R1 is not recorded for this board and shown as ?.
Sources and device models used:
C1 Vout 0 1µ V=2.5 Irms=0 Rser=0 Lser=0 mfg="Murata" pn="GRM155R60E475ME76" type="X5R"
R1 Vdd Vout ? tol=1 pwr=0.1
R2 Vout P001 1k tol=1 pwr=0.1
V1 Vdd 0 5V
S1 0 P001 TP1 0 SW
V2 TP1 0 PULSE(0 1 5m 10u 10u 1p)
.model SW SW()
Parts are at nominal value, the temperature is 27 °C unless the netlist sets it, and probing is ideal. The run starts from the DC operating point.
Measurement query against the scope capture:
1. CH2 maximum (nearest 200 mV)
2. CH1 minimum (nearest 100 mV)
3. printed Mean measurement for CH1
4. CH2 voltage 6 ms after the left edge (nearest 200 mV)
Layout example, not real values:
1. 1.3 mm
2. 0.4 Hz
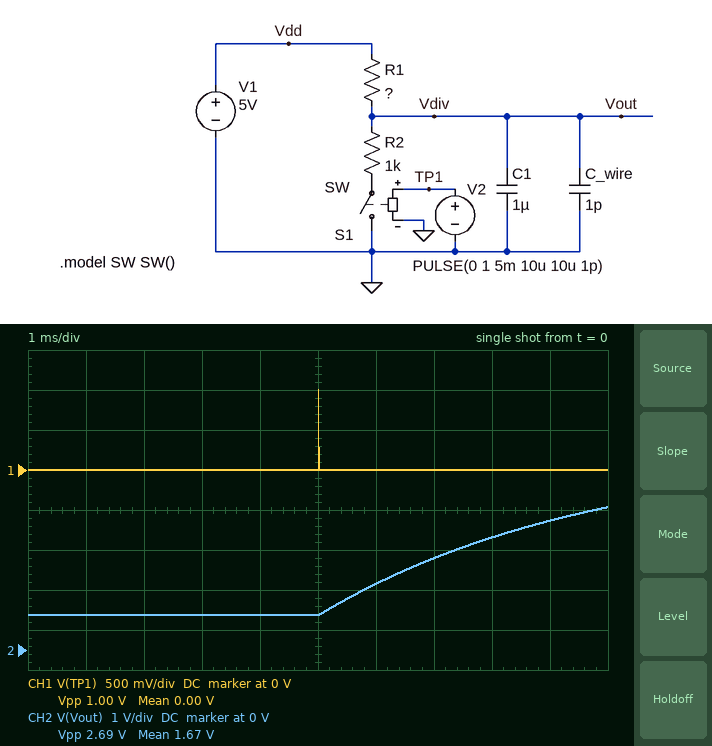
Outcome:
1. 3.6 V
2. 0 V
3. 0.00 V
4. 1.6 V
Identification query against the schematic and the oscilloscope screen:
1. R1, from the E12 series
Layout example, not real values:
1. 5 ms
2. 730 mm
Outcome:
1. 4.7 kΩ
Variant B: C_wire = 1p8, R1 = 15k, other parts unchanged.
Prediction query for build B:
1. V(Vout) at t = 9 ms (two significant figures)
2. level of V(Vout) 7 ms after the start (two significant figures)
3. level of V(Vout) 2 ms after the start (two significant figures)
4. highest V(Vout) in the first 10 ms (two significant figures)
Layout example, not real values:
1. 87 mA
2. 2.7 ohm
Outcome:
1. 1.4 V
2. 890 mV
3. 310 mV
4. 1.6 V
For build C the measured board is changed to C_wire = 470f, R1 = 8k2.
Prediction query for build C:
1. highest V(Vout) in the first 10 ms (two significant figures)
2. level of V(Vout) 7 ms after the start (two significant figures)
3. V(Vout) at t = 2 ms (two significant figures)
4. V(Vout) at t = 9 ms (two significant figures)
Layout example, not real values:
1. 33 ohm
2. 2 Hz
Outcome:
1. 2.6 V
2. 1.5 V
3. 540 mV
4. 2.3 V
